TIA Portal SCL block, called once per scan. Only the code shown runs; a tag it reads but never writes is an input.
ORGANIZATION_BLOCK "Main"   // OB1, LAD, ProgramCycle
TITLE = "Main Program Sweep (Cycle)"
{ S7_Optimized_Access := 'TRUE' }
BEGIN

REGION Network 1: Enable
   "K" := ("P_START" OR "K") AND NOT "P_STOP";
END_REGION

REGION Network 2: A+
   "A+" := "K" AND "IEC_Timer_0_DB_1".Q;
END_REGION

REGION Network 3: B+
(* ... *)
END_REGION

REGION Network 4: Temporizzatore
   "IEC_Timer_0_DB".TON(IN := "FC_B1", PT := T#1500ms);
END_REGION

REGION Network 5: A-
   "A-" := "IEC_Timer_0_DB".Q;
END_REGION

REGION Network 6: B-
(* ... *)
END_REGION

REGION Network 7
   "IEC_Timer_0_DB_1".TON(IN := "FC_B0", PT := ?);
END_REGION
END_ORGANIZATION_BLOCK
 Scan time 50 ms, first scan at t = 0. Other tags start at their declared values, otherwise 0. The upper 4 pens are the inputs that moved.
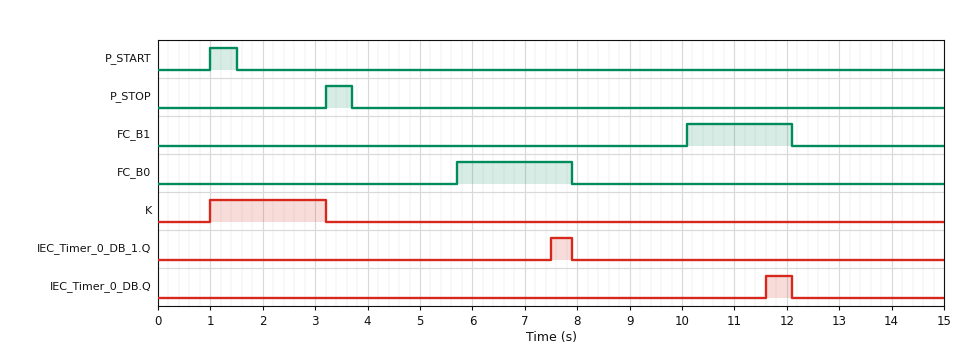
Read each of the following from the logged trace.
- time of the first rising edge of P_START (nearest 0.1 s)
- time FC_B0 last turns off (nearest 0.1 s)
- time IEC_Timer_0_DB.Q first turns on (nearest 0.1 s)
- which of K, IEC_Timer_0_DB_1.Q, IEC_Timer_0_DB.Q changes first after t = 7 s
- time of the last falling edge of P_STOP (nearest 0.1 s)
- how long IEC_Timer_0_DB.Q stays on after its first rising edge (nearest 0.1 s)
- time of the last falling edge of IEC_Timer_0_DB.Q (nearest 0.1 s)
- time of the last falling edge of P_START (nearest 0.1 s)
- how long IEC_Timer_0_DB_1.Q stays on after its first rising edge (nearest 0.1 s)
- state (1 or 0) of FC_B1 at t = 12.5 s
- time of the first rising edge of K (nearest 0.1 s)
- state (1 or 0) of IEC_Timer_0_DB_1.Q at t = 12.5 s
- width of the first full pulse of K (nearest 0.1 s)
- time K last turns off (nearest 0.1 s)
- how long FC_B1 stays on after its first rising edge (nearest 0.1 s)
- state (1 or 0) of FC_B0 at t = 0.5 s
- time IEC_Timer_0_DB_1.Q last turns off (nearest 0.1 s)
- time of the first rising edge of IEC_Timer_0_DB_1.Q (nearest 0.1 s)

1.0 s
7.9 s
11.6 s
IEC_Timer_0_DB_1.Q
3.7 s
0.5 s
12.1 s
1.5 s
0.4 s
0
1.0 s
0
2.2 s
3.2 s
2.0 s
0
7.9 s
7.5 s
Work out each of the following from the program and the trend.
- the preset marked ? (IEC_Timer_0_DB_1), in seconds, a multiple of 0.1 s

1.8 s
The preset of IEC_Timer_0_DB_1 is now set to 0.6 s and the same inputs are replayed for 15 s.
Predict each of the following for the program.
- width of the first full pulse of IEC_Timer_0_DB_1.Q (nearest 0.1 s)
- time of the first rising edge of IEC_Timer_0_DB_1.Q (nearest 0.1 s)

1.6 s
6.3 s
